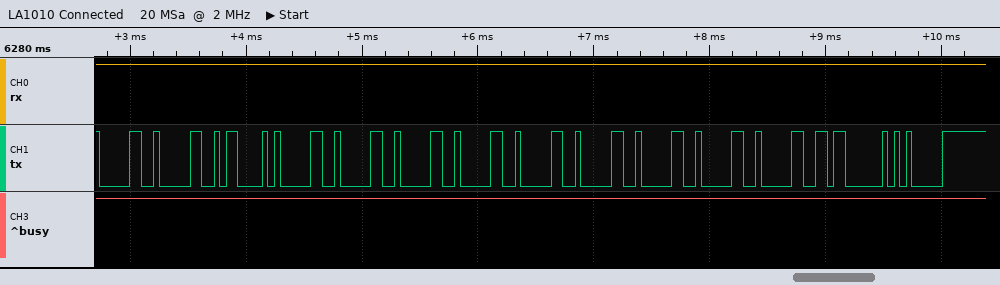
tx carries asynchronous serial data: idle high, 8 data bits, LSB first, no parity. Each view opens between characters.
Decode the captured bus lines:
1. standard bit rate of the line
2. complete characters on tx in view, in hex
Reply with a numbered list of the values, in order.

1. 19200 baud
2. 30, 30, 43, 30, 30, 30, 30, 30, 30, 30, 30, 30, 03, 05
